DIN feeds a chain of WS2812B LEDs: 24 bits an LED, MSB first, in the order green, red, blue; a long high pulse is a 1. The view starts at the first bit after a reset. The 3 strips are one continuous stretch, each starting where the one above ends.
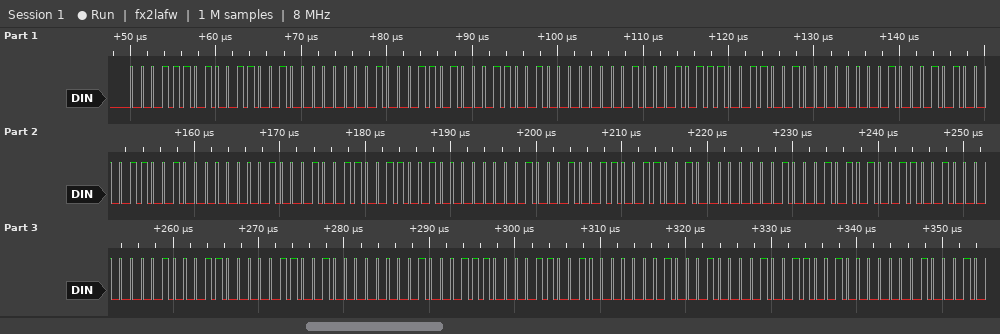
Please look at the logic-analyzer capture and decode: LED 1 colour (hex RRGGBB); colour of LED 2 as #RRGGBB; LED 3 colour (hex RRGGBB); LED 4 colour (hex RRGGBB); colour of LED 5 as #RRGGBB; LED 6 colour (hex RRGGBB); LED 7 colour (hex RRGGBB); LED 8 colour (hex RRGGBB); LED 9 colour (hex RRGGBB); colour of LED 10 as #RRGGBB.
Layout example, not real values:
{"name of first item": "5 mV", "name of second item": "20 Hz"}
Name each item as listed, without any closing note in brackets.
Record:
{"LED 1 colour": "#321D01", "colour of LED 2 as #RRGGBB": "#321A01", "LED 3 colour": "#321701", "LED 4 colour": "#321401", "colour of LED 5 as #RRGGBB": "#321301", "LED 6 colour": "#321301", "LED 7 colour": "#321501", "LED 8 colour": "#321801", "LED 9 colour": "#321C02", "colour of LED 10 as #RRGGBB": "#322102"}
